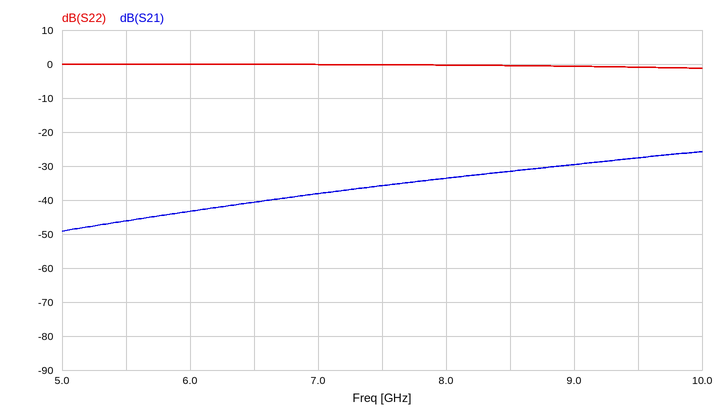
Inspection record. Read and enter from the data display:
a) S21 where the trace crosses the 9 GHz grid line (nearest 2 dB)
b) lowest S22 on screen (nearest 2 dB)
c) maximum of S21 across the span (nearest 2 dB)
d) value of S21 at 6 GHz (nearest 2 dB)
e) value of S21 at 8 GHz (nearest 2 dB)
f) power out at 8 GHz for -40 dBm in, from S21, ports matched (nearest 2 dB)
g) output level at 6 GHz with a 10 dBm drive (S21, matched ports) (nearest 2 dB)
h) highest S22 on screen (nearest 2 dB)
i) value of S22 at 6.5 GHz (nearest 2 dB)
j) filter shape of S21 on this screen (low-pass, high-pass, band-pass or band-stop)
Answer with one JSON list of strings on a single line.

["-30 dB", "-2 dB", "-26 dB", "-44 dB", "-34 dB", "-74 dBm", "-34 dBm", "0 dB", "0 dB", "high-pass"]
